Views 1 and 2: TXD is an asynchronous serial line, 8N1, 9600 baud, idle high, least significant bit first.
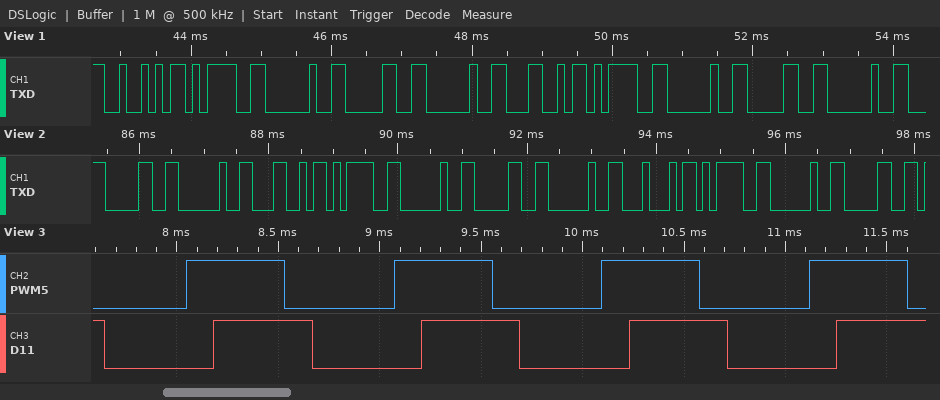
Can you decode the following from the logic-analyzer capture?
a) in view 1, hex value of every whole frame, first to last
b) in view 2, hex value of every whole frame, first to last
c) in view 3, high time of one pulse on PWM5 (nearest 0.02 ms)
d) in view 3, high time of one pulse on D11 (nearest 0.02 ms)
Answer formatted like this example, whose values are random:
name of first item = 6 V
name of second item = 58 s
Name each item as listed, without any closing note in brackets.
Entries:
in view 1, hex value of every whole frame, first to last = 0x52 0x3D 0x20 0x30 0x20 0x4C 0x3D 0x20 0x30 0x20
in view 2, hex value of every whole frame, first to last = 30 20 4C 3D 20 30 20 44 3D 20 30
in view 3, high time of one pulse on PWM5 = 0.48 ms
in view 3, high time of one pulse on D11 = 0.48 ms
